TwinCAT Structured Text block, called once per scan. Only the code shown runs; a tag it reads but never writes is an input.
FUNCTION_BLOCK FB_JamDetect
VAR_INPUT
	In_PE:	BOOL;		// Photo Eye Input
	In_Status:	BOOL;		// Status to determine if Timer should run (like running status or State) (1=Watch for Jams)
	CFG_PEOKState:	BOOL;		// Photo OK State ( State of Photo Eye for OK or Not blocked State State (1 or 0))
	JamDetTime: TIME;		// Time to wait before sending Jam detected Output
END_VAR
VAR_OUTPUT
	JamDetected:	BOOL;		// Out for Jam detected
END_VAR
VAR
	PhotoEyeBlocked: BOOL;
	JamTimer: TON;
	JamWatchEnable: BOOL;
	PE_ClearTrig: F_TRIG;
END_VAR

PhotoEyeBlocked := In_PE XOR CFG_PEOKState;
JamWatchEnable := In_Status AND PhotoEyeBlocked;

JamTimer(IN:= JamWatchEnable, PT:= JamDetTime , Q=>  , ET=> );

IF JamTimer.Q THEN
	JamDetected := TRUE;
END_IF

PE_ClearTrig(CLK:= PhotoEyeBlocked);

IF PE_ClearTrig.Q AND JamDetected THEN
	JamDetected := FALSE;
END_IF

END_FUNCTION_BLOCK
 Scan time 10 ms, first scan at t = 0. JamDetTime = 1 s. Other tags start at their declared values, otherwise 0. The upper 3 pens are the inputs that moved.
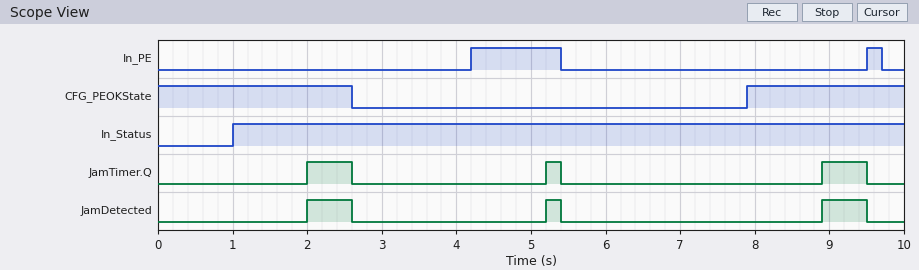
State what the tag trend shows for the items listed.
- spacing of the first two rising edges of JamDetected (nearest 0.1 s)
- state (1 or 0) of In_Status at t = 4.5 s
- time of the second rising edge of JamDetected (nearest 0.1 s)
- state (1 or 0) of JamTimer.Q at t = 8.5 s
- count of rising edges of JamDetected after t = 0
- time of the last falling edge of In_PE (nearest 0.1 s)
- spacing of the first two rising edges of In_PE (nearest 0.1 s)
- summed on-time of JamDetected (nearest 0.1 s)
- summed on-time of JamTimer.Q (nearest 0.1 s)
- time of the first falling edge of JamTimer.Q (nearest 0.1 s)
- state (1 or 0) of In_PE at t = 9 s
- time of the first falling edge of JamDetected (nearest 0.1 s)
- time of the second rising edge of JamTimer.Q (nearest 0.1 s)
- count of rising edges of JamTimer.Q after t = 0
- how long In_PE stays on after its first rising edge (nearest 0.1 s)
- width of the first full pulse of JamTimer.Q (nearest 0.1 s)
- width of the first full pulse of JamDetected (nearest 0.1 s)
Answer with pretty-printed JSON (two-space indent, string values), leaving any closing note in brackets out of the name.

{
  "spacing of the first two rising edges of JamDetected": "3.2 s",
  "state (1 or 0) of In_Status at t = 4.5 s": "1",
  "time of the second rising edge of JamDetected": "5.2 s",
  "state (1 or 0) of JamTimer.Q at t = 8.5 s": "0",
  "count of rising edges of JamDetected after t = 0": "3",
  "time of the last falling edge of In_PE": "9.7 s",
  "spacing of the first two rising edges of In_PE": "5.3 s",
  "summed on-time of JamDetected": "1.4 s",
  "summed on-time of JamTimer.Q": "1.4 s",
  "time of the first falling edge of JamTimer.Q": "2.6 s",
  "state (1 or 0) of In_PE at t = 9 s": "0",
  "time of the first falling edge of JamDetected": "2.6 s",
  "time of the second rising edge of JamTimer.Q": "5.2 s",
  "count of rising edges of JamTimer.Q after t = 0": "3",
  "how long In_PE stays on after its first rising edge": "1.2 s",
  "width of the first full pulse of JamTimer.Q": "0.6 s",
  "width of the first full pulse of JamDetected": "0.6 s"
}
